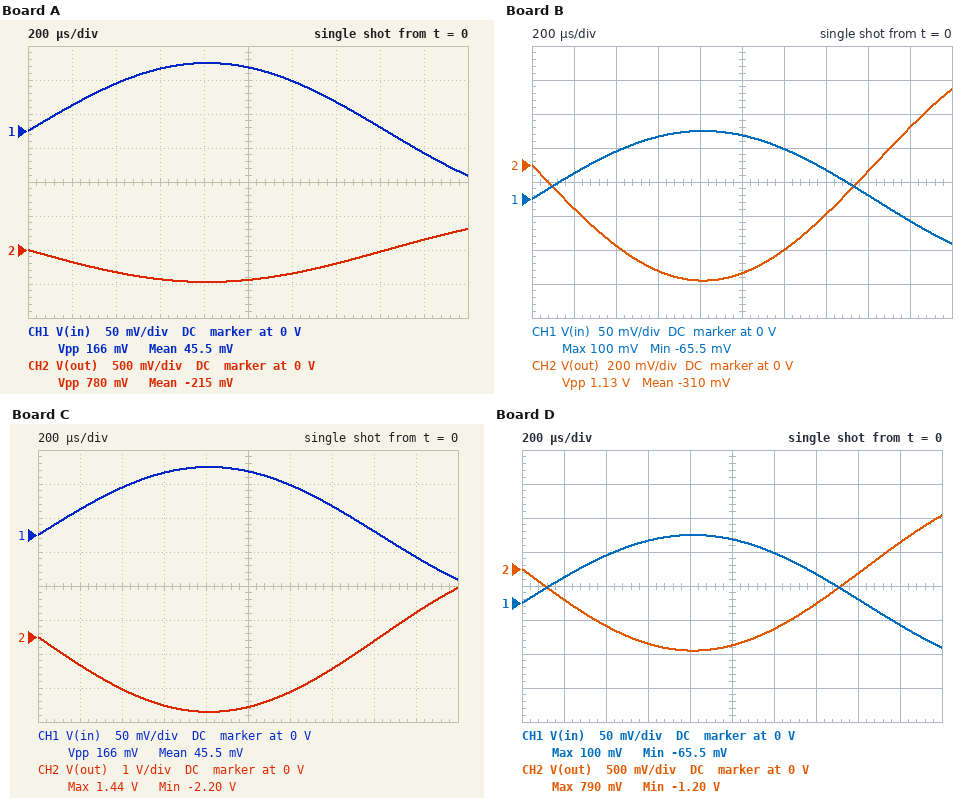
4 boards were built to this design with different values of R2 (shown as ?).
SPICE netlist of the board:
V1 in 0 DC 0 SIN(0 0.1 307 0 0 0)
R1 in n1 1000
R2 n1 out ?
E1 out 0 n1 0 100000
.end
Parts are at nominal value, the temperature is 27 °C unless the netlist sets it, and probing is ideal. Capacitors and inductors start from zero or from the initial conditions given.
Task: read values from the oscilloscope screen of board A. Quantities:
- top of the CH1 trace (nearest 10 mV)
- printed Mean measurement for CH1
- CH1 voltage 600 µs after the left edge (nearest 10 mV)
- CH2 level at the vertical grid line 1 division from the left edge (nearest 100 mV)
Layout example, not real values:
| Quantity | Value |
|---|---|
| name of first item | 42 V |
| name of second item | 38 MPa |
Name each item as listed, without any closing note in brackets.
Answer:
| Quantity | Value |
|---|---|
| top of the CH1 trace | 100 mV |
| printed Mean measurement for CH1 | 45.5 mV |
| CH1 voltage 600 µs after the left edge | 90 mV |
| CH2 level at the vertical grid line 1 division from the left edge | -200 mV |
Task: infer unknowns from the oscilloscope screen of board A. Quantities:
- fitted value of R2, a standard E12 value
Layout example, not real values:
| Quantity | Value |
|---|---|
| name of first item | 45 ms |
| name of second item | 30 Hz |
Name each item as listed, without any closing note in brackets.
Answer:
| Quantity | Value |
|---|---|
| fitted value of R2, a standard E12 value | 4.7 kΩ |
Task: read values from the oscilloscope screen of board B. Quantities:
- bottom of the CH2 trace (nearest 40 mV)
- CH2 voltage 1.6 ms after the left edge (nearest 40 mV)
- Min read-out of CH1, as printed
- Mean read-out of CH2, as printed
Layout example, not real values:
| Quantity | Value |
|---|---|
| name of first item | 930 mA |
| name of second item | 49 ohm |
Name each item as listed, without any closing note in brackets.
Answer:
| Quantity | Value |
|---|---|
| bottom of the CH2 trace | -680 mV |
| CH2 voltage 1.6 ms after the left edge | -40 mV |
| Min read-out of CH1, as printed | -65.5 mV |
| Mean read-out of CH2, as printed | -310 mV |
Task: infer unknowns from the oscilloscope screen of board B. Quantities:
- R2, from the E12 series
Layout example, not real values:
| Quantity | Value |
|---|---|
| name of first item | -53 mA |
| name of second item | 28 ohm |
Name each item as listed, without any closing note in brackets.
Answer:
| Quantity | Value |
|---|---|
| R2, from the E12 series | 6.8 kΩ |
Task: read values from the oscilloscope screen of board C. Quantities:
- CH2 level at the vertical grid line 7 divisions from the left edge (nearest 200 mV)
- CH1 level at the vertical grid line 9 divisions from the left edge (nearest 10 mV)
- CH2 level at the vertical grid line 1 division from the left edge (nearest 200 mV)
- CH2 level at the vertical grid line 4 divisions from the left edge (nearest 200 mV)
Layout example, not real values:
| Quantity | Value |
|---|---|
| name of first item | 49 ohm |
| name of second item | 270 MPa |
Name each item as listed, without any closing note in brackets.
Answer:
| Quantity | Value |
|---|---|
| CH2 level at the vertical grid line 7 divisions from the left edge | -1.0 V |
| CH1 level at the vertical grid line 9 divisions from the left edge | -30 mV |
| CH2 level at the vertical grid line 1 division from the left edge | -800 mV |
| CH2 level at the vertical grid line 4 divisions from the left edge | -2.2 V |
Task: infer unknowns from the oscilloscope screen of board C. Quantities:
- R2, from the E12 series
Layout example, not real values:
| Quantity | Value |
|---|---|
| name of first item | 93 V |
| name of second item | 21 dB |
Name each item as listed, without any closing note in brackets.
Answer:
| Quantity | Value |
|---|---|
| R2, from the E12 series | 22 kΩ |
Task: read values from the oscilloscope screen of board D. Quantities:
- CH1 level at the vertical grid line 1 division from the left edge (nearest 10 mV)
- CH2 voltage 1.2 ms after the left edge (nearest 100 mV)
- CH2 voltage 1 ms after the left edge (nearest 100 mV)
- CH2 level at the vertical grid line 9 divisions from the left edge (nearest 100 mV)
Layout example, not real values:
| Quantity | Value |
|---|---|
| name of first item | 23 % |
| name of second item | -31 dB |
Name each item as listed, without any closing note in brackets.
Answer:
| Quantity | Value |
|---|---|
| CH1 level at the vertical grid line 1 division from the left edge | 40 mV |
| CH2 voltage 1.2 ms after the left edge | -900 mV |
| CH2 voltage 1 ms after the left edge | -1.1 V |
| CH2 level at the vertical grid line 9 divisions from the left edge | 400 mV |
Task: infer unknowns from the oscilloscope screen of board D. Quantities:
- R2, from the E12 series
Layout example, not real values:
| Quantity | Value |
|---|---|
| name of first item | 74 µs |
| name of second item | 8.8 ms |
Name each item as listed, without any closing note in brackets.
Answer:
| Quantity | Value |
|---|---|
| R2, from the E12 series | 12 kΩ |
